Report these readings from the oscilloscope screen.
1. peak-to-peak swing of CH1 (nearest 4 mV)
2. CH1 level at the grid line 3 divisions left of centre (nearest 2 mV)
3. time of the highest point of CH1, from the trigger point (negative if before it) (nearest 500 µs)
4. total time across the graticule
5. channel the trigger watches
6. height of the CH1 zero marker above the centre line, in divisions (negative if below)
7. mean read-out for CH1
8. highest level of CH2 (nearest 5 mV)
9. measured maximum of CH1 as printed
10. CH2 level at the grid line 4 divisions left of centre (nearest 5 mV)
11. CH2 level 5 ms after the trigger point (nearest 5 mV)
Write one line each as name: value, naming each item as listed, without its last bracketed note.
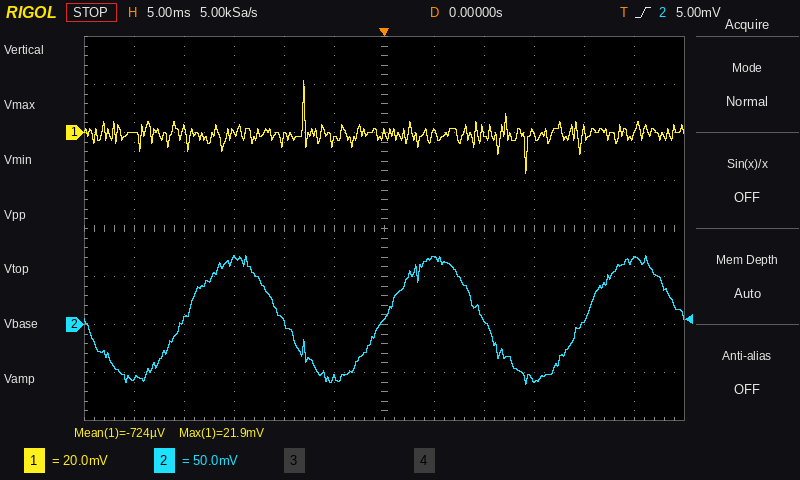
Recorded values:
peak-to-peak swing of CH1: 40 mV
CH1 level at the grid line 3 divisions left of centre: 0 mV
time of the highest point of CH1, from the trigger point (negative if before it): -8.0 ms
total time across the graticule: 60 ms
channel the trigger watches: CH2
height of the CH1 zero marker above the centre line, in divisions: +2.0 div
mean read-out for CH1: -724 µV
highest level of CH2: 70 mV
measured maximum of CH1 as printed: 21.9 mV
CH2 level at the grid line 4 divisions left of centre: 5 mV
CH2 level 5 ms after the trigger point: 70 mV
